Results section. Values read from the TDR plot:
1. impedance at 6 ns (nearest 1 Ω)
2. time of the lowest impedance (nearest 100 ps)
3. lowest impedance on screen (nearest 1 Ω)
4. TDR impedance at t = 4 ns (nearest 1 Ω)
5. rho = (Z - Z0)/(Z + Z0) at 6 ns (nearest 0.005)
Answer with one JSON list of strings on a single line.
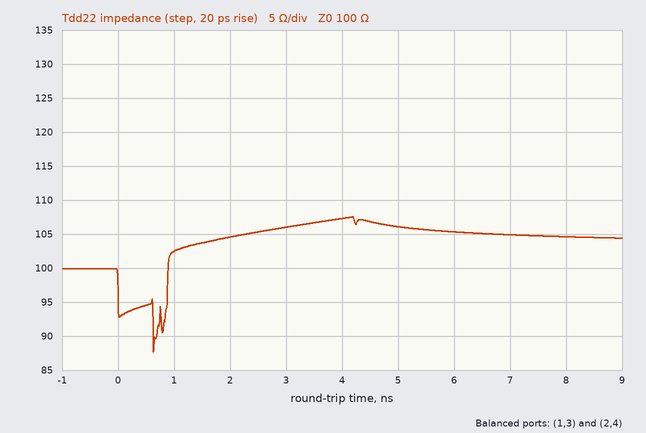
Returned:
["105 Ω", "600 ps", "88 Ω", "107 Ω", "+0.025"]
